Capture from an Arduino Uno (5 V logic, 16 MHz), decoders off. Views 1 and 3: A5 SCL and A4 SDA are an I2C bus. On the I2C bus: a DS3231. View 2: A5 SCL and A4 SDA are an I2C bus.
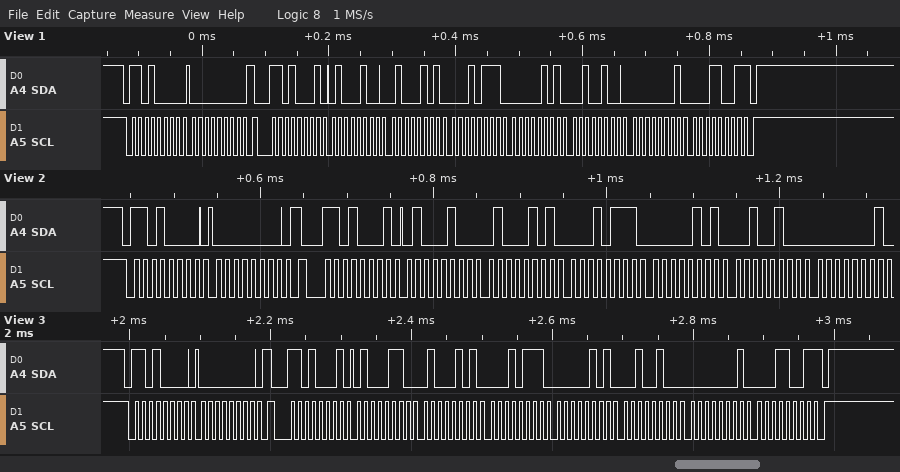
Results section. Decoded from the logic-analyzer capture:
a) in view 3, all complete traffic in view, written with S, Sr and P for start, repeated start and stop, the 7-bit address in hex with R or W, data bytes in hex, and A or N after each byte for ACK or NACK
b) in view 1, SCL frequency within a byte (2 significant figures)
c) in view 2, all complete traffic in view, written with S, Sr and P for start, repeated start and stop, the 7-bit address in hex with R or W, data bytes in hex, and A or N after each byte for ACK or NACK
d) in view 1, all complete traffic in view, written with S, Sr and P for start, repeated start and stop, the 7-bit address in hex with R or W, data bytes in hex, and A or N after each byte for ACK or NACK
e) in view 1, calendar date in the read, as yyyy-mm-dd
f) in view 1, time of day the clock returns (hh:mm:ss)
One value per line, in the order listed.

S 68W A 00 A Sr 68R A 46 A 45 A 17 A 05 A 24 A 01 A 19 N P
100 kHz
S 68W A 00 A Sr 68R A 44 A 45 A 17 A 05 A 24 A 01 A
S 68W A 00 A Sr 68R A 44 A 45 A 17 A 05 A 24 A 01 A 19 N P
2019-01-24
17:45:44
